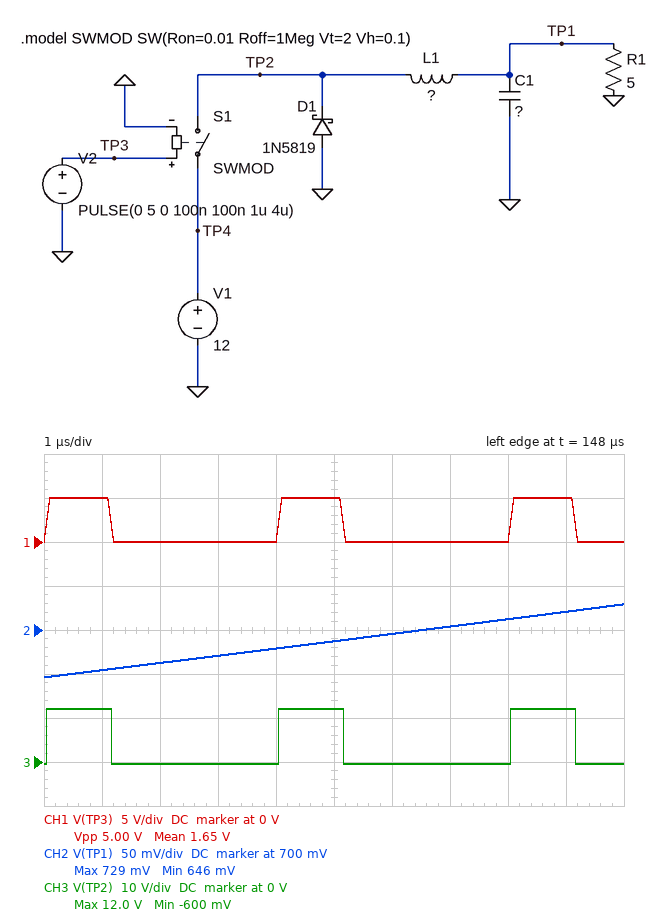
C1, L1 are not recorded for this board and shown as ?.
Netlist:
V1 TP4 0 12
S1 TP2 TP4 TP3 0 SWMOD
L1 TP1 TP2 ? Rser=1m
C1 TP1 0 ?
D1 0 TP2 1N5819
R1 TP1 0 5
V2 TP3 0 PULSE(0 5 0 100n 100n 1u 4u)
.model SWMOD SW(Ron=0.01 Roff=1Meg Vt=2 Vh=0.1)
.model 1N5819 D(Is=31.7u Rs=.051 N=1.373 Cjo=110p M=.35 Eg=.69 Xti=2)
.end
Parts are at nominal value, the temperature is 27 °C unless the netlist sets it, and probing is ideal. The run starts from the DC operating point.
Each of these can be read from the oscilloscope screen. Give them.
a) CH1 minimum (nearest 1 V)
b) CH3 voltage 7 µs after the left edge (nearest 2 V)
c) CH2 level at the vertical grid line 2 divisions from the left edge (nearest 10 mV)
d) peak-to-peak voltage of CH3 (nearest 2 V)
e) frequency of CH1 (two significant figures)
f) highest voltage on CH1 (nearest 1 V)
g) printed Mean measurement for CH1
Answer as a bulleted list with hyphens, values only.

- 0 V
- 0 V
- 660 mV
- 12 V
- 250 kHz
- 5 V
- 1.65 V
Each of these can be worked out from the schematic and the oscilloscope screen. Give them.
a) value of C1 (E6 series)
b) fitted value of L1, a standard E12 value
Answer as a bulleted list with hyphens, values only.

- 330 µF
- 150 µH
